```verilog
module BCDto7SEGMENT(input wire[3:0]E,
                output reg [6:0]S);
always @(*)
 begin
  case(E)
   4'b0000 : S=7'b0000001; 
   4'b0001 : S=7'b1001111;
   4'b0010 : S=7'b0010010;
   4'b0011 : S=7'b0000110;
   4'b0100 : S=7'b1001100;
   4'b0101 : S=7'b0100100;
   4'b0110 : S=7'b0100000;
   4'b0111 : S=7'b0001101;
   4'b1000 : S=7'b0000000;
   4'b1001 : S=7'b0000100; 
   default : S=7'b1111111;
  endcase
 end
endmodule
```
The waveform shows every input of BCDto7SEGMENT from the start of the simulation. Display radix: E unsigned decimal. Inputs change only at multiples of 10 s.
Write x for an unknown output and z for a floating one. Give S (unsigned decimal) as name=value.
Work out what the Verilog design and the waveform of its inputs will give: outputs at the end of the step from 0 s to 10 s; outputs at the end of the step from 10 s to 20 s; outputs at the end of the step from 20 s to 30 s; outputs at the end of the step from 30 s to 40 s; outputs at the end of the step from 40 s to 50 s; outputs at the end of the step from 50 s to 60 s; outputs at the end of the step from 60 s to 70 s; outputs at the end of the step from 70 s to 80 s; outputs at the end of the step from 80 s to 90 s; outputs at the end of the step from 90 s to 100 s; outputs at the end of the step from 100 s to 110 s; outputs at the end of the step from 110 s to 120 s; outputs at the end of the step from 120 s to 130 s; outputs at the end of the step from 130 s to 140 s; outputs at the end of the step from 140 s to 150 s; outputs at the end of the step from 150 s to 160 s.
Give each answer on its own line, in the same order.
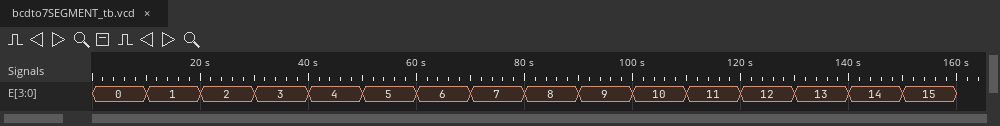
S=1
S=79
S=18
S=6
S=76
S=36
S=32
S=13
S=0
S=4
S=127
S=127
S=127
S=127
S=127
S=127
